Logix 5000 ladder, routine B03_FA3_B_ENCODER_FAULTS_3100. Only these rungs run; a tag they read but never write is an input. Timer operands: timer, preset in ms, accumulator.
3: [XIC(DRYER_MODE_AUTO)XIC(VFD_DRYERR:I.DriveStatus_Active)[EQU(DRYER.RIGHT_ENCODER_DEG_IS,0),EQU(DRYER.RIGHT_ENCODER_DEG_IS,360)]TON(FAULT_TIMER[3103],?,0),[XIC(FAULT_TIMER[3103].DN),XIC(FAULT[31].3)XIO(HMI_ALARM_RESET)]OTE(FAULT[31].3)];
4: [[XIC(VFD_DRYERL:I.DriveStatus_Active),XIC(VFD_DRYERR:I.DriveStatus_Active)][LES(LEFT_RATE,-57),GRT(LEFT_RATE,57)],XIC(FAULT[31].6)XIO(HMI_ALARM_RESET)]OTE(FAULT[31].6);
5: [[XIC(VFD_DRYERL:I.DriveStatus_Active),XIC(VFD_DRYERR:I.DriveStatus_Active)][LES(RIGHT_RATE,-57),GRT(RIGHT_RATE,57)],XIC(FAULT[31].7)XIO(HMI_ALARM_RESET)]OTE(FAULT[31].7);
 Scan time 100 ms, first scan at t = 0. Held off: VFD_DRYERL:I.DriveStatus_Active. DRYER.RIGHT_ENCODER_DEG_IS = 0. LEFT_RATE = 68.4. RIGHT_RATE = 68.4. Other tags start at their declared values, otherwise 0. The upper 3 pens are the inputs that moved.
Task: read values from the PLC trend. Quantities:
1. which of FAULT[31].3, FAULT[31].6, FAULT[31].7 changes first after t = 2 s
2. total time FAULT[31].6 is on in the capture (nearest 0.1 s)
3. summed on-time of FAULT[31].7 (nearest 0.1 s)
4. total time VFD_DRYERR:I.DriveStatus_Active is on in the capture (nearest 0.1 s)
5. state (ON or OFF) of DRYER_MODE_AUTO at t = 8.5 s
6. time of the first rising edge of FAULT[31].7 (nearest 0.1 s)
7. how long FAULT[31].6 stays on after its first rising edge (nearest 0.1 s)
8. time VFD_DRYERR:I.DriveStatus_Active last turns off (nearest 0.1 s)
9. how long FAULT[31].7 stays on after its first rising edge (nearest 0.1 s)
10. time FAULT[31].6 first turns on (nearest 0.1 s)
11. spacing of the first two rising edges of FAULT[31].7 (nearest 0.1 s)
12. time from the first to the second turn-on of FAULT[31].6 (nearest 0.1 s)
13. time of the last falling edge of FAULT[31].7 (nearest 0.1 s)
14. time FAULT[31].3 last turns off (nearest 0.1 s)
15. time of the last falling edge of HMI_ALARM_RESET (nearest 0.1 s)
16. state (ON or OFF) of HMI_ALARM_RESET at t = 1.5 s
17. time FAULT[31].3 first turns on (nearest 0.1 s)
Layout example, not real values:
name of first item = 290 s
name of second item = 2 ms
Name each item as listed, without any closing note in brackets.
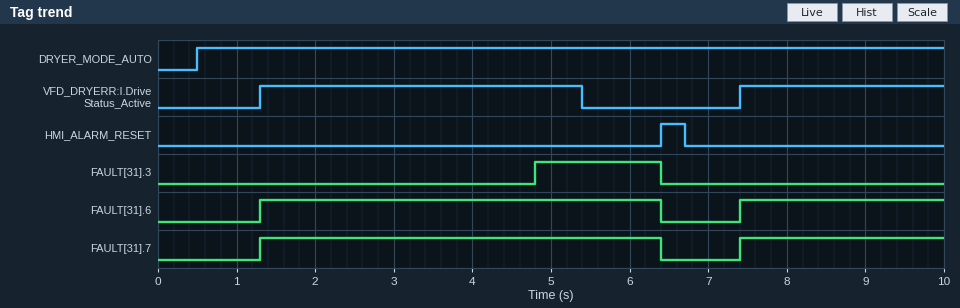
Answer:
which of FAULT[31].3, FAULT[31].6, FAULT[31].7 changes first after t = 2 s = FAULT[31].3
total time FAULT[31].6 is on in the capture = 7.7 s
summed on-time of FAULT[31].7 = 7.7 s
total time VFD_DRYERR:I.DriveStatus_Active is on in the capture = 6.7 s
state (ON or OFF) of DRYER_MODE_AUTO at t = 8.5 s = ON
time of the first rising edge of FAULT[31].7 = 1.3 s
how long FAULT[31].6 stays on after its first rising edge = 5.1 s
time VFD_DRYERR:I.DriveStatus_Active last turns off = 5.4 s
how long FAULT[31].7 stays on after its first rising edge = 5.1 s
time FAULT[31].6 first turns on = 1.3 s
spacing of the first two rising edges of FAULT[31].7 = 6.1 s
time from the first to the second turn-on of FAULT[31].6 = 6.1 s
time of the last falling edge of FAULT[31].7 = 6.4 s
time FAULT[31].3 last turns off = 6.4 s
time of the last falling edge of HMI_ALARM_RESET = 6.7 s
state (ON or OFF) of HMI_ALARM_RESET at t = 1.5 s = OFF
time FAULT[31].3 first turns on = 4.8 s
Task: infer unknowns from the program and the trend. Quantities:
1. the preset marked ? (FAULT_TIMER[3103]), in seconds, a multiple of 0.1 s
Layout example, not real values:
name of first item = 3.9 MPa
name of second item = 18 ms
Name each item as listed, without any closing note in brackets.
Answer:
the preset marked ? (FAULT_TIMER[3103]), in seconds, a multiple of 0.1 s = 3.5 s
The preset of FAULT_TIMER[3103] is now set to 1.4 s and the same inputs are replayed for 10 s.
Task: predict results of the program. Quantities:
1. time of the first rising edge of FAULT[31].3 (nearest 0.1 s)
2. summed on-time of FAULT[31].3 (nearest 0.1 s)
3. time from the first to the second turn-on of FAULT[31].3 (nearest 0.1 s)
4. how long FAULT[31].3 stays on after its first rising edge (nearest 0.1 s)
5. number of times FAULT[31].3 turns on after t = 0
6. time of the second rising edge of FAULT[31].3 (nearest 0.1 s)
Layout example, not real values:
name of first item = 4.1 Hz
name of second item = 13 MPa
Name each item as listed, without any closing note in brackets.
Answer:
time of the first rising edge of FAULT[31].3 = 2.7 s
summed on-time of FAULT[31].3 = 4.9 s
time from the first to the second turn-on of FAULT[31].3 = 6.1 s
how long FAULT[31].3 stays on after its first rising edge = 3.7 s
number of times FAULT[31].3 turns on after t = 0 = 2
time of the second rising edge of FAULT[31].3 = 8.8 s
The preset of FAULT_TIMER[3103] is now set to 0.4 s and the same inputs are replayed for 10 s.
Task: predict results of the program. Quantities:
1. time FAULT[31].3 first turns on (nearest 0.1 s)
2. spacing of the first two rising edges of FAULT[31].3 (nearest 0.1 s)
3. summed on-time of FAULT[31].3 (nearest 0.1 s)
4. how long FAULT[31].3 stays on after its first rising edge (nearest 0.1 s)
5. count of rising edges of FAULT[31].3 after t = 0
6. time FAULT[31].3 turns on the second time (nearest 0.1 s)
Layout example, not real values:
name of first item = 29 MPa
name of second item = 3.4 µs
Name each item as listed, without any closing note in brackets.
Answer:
time FAULT[31].3 first turns on = 1.7 s
spacing of the first two rising edges of FAULT[31].3 = 6.1 s
summed on-time of FAULT[31].3 = 6.9 s
how long FAULT[31].3 stays on after its first rising edge = 4.7 s
count of rising edges of FAULT[31].3 after t = 0 = 2
time FAULT[31].3 turns on the second time = 7.8 s
